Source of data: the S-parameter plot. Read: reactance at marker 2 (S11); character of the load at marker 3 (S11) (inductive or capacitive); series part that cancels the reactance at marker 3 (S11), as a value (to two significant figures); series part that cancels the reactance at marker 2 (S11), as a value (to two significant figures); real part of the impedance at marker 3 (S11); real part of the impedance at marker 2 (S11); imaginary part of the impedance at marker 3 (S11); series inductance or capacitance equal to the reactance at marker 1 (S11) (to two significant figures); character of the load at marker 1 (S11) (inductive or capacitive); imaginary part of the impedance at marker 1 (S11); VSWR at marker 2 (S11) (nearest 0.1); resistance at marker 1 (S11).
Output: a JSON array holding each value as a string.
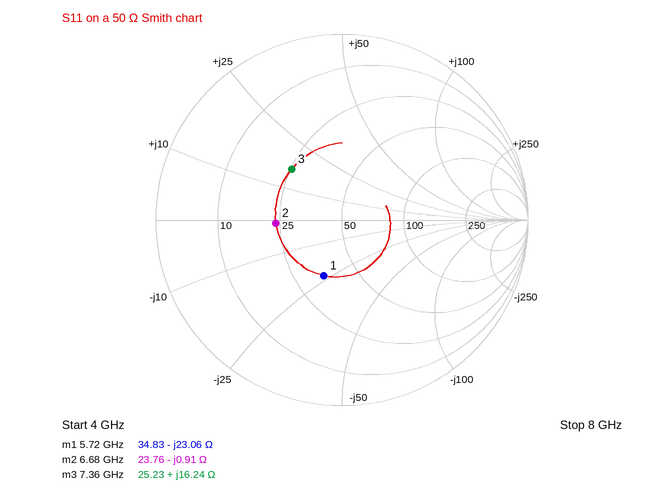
["-0.91 Ω", "inductive", "1.3 pF", "22 pH", "25.23 Ω", "23.76 Ω", "+16.24 Ω", "1.2 pF", "capacitive", "-23.06 Ω", "2.1", "34.83 Ω"]
